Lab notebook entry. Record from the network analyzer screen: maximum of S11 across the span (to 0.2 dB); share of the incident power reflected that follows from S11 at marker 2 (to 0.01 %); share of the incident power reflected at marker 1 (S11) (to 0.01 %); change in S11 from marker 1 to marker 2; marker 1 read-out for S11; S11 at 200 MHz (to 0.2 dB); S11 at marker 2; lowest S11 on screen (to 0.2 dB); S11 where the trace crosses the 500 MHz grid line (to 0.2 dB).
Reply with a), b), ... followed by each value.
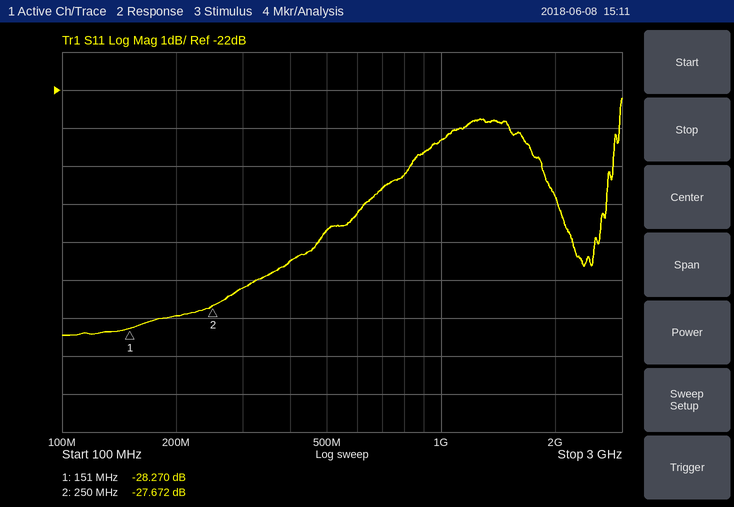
a) -22.2 dB
b) 0.17 %
c) 0.15 %
d) 0.598 dB
e) -28.270 dB
f) -28.0 dB
g) -27.672 dB
h) -28.4 dB
i) -25.6 dB
